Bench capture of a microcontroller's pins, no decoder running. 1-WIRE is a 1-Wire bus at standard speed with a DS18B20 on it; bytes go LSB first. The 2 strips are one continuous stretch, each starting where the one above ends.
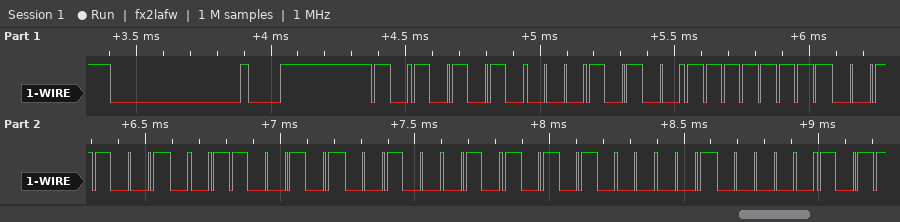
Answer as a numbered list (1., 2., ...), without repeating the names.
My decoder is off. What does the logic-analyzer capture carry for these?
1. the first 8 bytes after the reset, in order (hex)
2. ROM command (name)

1. 55 28 FF 4C A6 44 15 04
2. Match ROM
